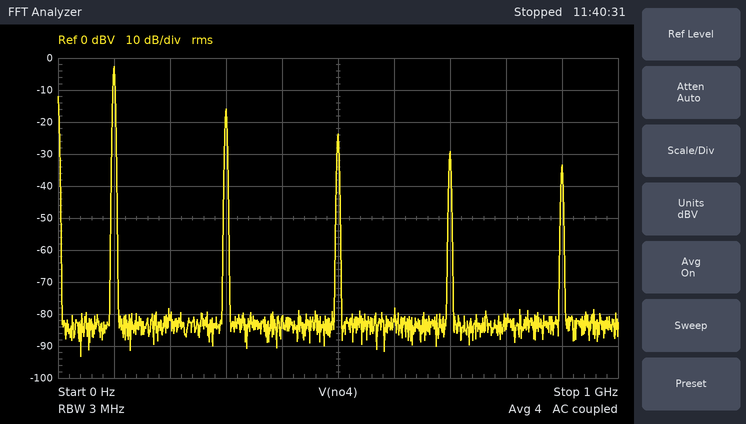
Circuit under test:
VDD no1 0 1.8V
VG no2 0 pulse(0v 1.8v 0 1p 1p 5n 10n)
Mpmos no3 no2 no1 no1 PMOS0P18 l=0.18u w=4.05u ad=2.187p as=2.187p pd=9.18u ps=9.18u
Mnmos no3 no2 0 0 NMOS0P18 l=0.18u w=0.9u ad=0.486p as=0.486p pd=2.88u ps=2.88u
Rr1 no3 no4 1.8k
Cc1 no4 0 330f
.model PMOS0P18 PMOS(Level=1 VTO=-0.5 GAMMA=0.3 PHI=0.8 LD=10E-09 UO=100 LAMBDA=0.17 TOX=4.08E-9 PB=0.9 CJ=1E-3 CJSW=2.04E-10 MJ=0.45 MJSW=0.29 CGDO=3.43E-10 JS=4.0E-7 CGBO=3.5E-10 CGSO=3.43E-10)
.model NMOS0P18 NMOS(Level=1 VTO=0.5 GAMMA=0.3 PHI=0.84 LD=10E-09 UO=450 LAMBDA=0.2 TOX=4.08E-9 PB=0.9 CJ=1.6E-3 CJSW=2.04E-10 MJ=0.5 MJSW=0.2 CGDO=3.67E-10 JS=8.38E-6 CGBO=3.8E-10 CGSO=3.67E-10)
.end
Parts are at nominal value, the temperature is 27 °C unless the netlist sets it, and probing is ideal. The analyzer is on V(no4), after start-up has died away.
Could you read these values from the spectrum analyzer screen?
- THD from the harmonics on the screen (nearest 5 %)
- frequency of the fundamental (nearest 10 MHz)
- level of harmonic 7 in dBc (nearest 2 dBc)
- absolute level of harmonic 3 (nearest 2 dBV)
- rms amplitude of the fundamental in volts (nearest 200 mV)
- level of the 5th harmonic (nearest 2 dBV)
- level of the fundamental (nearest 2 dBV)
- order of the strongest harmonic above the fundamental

25 %
100 MHz
-26 dBc
-16 dBV
800 mV
-24 dBV
-2 dBV
3
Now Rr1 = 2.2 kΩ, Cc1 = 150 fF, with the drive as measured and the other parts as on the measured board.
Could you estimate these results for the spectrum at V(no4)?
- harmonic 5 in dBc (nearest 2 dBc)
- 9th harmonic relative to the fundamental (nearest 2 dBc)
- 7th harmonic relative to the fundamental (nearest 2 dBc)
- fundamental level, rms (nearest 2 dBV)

-18 dBc
-26 dBc
-22 dBc
-2 dBV
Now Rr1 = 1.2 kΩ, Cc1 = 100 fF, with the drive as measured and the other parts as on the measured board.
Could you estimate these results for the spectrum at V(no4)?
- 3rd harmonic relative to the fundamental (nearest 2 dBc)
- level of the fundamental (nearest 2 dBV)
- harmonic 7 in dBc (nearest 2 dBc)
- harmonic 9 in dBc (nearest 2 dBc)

-10 dBc
-2 dBV
-18 dBc
-22 dBc
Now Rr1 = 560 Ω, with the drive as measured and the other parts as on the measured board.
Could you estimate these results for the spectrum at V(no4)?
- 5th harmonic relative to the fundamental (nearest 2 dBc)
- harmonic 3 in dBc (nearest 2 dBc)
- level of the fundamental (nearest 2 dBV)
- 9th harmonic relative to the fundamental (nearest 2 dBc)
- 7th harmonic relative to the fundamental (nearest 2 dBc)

-16 dBc
-10 dBc
-2 dBV
-26 dBc
-22 dBc
